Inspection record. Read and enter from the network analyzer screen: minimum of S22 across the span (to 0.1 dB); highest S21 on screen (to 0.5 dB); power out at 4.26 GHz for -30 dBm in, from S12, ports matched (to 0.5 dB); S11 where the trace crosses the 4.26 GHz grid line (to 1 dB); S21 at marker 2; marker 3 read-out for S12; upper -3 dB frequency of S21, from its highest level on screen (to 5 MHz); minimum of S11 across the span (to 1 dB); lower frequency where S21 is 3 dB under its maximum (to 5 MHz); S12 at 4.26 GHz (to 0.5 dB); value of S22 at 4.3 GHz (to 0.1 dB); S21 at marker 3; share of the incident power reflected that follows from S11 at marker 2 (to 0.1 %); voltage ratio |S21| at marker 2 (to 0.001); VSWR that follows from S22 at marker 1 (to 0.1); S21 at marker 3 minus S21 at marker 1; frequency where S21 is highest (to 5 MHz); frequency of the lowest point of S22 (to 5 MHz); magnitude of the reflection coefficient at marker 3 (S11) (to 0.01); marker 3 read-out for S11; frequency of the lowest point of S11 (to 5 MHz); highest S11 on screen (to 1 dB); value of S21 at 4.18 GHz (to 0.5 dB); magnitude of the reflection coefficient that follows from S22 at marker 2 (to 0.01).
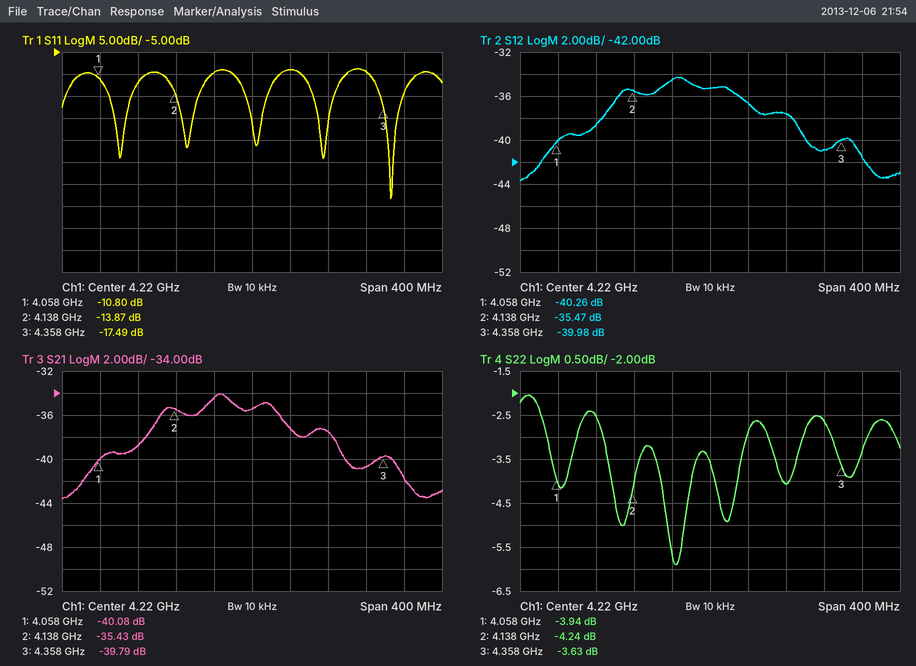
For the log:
-5.9 dB
-34.0 dB
-66.5 dBm
-9 dB
-35.43 dB
-39.98 dB
4.260 GHz
-38 dB
4.115 GHz
-36.5 dB
-4.1 dB
-39.79 dB
4.1 %
0.017
4.5
0.29 dB
4.185 GHz
4.185 GHz
0.13
-17.49 dB
4.365 GHz
-9 dB
-34.5 dB
0.61
